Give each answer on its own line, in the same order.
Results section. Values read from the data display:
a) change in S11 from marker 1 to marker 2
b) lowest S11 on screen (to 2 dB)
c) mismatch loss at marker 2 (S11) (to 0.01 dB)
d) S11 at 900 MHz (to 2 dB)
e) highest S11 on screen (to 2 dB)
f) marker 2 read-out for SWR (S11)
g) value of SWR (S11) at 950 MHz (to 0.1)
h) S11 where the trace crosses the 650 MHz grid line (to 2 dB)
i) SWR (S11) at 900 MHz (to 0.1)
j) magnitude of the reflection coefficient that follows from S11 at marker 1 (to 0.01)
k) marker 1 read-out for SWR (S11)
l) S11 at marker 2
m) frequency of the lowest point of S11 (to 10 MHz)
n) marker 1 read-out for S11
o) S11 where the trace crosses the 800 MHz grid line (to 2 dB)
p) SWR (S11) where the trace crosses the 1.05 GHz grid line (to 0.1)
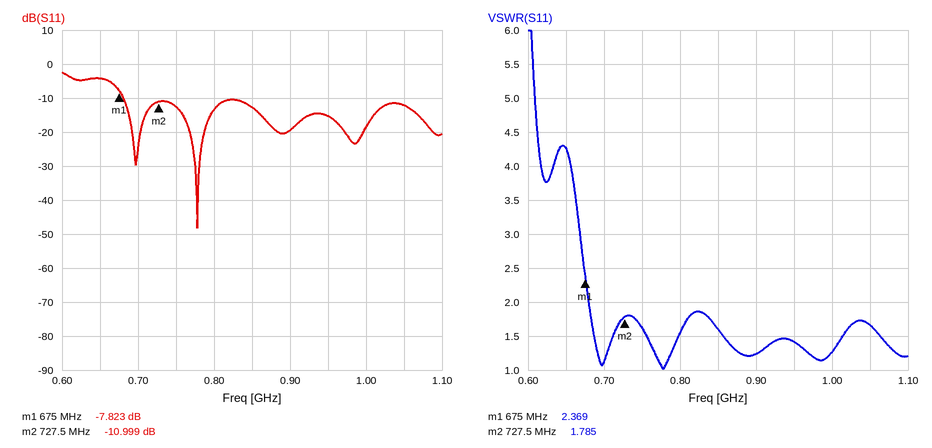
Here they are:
-3.176 dB
-48 dB
0.36 dB
-20 dB
-2 dB
1.785
1.4
-4 dB
1.2
0.41
2.369
-10.999 dB
780 MHz
-7.823 dB
-14 dB
1.7
